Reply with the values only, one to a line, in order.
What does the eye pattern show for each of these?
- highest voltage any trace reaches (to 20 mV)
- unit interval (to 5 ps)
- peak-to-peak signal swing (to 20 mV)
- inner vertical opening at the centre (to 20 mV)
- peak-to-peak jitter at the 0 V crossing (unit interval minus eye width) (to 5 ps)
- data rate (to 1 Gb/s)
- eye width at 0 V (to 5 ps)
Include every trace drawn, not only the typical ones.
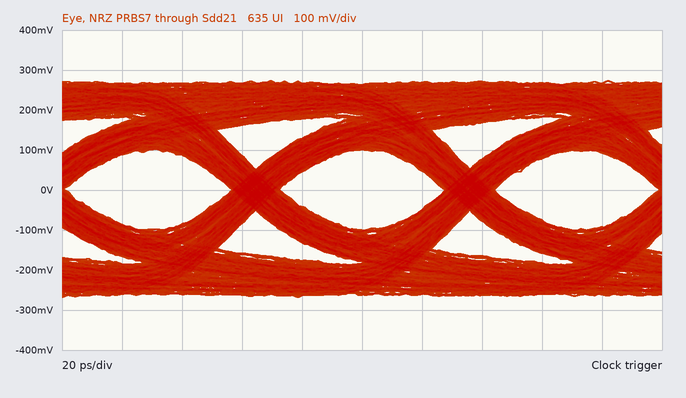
280 mV
70 ps
540 mV
200 mV
15 ps
14 Gb/s
55 ps
